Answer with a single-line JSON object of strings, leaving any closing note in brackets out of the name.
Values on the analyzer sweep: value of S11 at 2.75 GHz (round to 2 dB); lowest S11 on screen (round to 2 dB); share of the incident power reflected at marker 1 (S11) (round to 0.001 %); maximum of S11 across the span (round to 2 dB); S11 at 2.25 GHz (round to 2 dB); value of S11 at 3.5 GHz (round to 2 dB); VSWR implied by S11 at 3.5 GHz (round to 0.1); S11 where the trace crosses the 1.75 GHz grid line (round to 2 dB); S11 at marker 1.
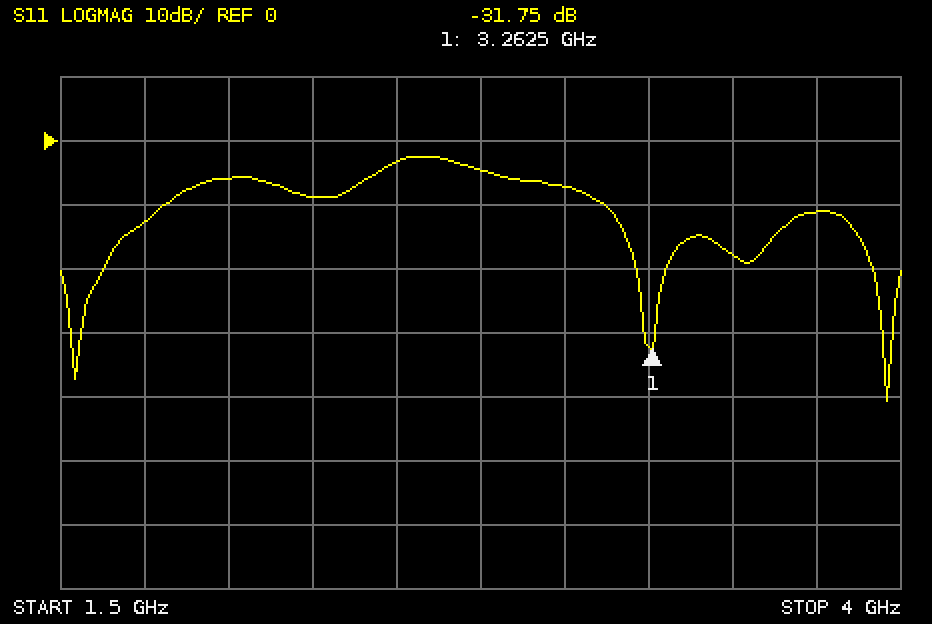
{"value of S11 at 2.75 GHz": "-4 dB", "lowest S11 on screen": "-40 dB", "share of the incident power reflected at marker 1 (S11)": "0.067 %", "maximum of S11 across the span": "-2 dB", "S11 at 2.25 GHz": "-8 dB", "value of S11 at 3.5 GHz": "-18 dB", "VSWR implied by S11 at 3.5 GHz": "1.3", "S11 where the trace crosses the 1.75 GHz grid line": "-12 dB", "S11 at marker 1": "-31.75 dB"}
